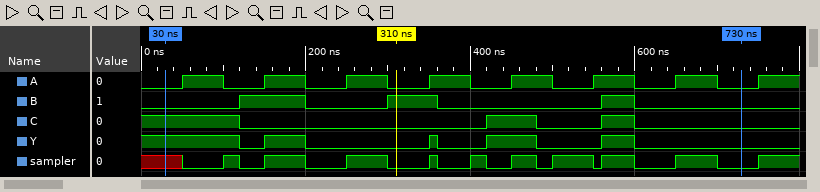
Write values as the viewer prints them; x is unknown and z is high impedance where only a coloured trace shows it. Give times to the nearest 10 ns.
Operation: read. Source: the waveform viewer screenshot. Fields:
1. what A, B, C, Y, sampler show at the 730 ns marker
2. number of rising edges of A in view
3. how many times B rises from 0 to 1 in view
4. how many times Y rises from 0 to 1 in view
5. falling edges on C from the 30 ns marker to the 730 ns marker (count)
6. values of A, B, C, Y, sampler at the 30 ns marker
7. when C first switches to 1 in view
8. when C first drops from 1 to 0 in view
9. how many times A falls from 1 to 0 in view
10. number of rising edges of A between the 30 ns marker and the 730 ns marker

A=0, B=0, C=0, Y=0, sampler=0
8
3
4
3
A=0, B=0, C=1, Y=1, sampler=x
420 ns
120 ns
7
7
